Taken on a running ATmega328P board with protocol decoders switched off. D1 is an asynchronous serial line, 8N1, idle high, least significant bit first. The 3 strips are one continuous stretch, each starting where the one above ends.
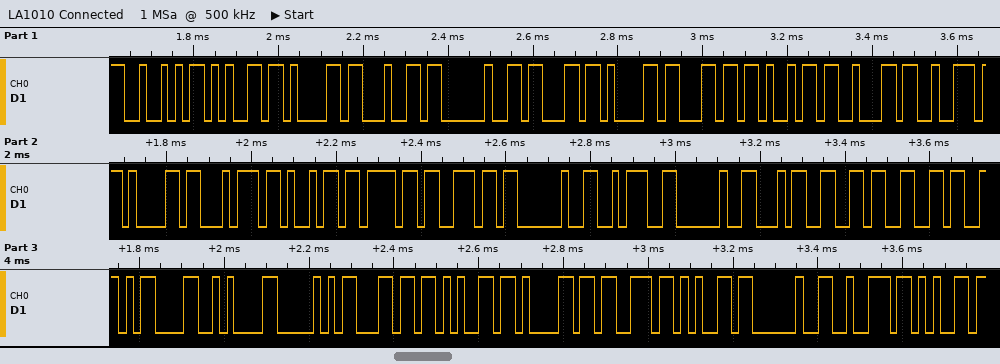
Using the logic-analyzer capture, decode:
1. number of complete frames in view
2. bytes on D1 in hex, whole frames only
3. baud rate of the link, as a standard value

33
52 65 61 64 20 63 61 6C 69 62 72 61 74 69 6F 6E 20 3A 20 34 36 36 0D 0A 50 6C 65 61 73 65 20 72 65
57600 baud
